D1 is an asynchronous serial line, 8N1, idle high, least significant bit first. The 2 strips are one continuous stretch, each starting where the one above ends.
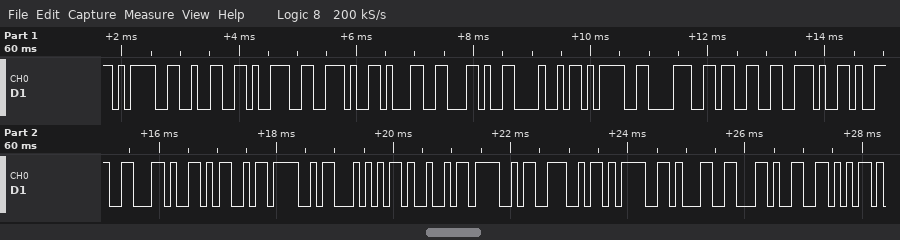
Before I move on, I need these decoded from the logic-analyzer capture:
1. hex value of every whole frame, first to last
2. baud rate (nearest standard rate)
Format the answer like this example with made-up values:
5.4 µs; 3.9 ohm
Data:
3D 32 39 2E 31 2C 48 3D 38 33 2E 39 2C 4D 4F 54 49 4F 4E 3D 31 2C 56; 9600 baud
